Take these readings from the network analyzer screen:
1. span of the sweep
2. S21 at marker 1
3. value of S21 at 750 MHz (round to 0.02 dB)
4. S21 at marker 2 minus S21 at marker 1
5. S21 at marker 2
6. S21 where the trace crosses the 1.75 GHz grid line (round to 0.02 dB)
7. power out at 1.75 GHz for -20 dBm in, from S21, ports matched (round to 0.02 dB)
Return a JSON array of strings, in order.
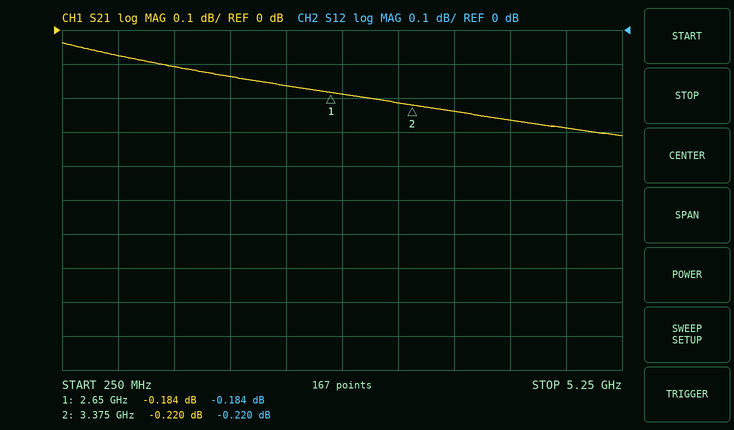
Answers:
["5 GHz", "-0.184 dB", "-0.08 dB", "-0.036 dB", "-0.220 dB", "-0.14 dB", "-20.14 dBm"]
